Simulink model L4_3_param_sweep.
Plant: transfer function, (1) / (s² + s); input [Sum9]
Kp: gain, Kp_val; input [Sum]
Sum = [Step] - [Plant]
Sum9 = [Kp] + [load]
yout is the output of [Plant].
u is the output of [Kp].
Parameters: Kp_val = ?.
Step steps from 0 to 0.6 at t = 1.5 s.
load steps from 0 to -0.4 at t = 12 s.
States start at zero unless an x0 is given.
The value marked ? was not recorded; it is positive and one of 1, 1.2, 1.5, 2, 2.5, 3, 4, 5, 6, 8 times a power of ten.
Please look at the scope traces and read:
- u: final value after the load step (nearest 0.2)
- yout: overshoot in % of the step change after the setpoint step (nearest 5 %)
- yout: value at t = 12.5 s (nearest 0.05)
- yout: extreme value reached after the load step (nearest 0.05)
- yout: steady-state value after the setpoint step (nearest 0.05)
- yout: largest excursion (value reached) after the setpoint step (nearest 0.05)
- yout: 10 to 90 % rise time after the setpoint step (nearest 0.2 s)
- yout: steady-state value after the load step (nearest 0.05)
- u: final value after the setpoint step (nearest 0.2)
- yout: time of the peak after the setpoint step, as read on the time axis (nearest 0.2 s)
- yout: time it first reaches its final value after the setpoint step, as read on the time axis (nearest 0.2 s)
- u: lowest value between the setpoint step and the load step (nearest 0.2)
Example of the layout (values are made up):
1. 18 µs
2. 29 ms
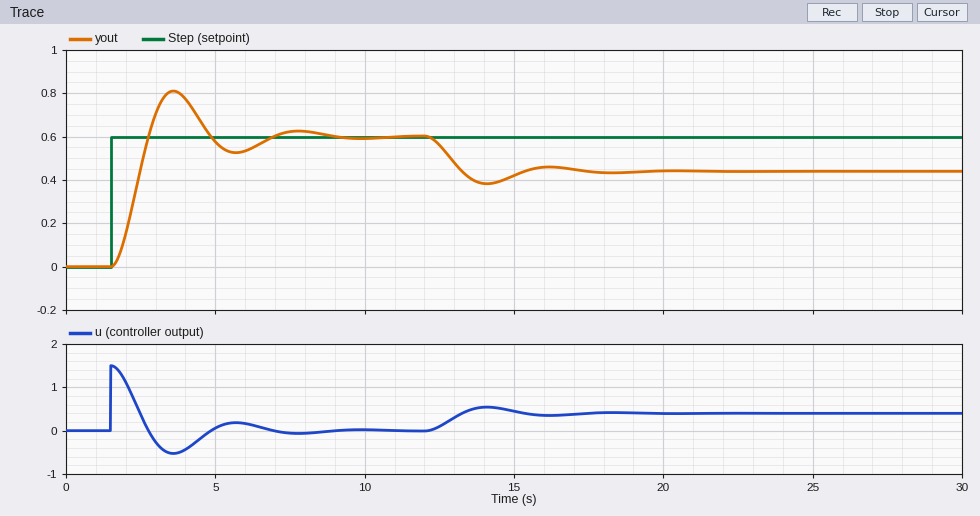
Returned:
1. 0.4
2. 35 %
3. 0.55
4. 0.40
5. 0.60
6. 0.80
7. 0.8 s
8. 0.45
9. 0.0
10. 3.6 s
11. 2.8 s
12. -0.6
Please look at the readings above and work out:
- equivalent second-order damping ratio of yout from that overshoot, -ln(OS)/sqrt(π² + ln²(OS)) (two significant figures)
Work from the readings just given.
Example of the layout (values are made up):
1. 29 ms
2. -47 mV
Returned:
1. 0.32
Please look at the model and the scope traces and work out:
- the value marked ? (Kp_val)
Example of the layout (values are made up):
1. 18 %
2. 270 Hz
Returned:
1. 2.5
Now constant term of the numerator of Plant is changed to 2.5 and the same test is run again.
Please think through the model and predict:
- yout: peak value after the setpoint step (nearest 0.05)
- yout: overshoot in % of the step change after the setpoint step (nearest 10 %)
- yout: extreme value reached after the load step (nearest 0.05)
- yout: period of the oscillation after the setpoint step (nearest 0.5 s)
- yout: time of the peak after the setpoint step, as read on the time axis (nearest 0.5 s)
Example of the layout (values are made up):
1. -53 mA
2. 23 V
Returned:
1. 0.90
2. 50 %
3. 0.35
4. 2.5 s
5. 3.0 s
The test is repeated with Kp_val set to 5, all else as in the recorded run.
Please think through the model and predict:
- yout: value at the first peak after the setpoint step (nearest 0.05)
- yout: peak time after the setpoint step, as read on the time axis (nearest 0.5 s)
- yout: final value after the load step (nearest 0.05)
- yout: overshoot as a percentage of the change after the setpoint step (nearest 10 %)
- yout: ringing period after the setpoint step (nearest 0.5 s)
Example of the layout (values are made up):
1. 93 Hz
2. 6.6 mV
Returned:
1. 0.90
2. 3.0 s
3. 0.50
4. 50 %
5. 3.0 s
